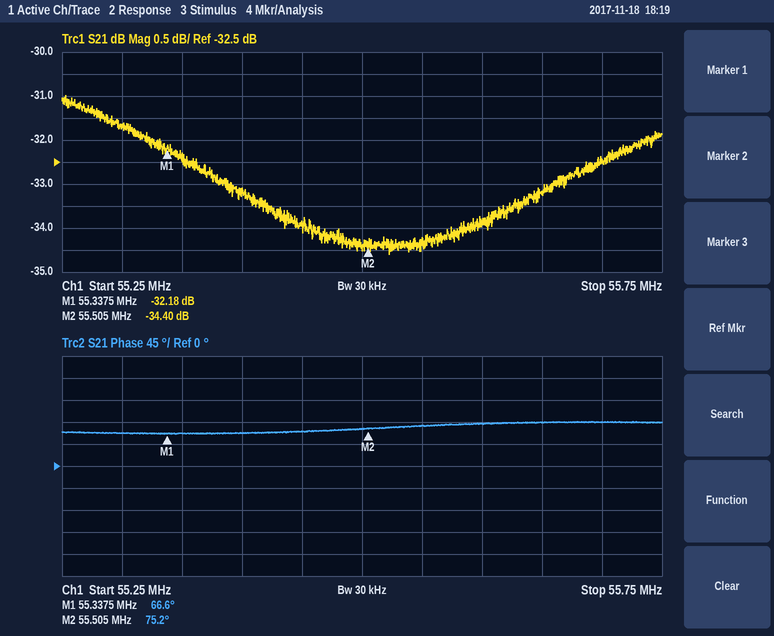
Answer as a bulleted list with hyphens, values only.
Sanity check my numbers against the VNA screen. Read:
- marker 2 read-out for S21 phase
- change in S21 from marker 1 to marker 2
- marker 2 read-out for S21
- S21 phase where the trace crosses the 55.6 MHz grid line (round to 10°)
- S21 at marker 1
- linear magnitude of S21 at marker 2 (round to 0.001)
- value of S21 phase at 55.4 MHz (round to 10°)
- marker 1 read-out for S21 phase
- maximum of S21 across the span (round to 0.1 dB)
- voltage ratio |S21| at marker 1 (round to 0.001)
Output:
- 75.2°
- -2.22 dB
- -34.40 dB
- 90°
- -32.18 dB
- 0.019
- 70°
- 66.6°
- -31.0 dB
- 0.025
